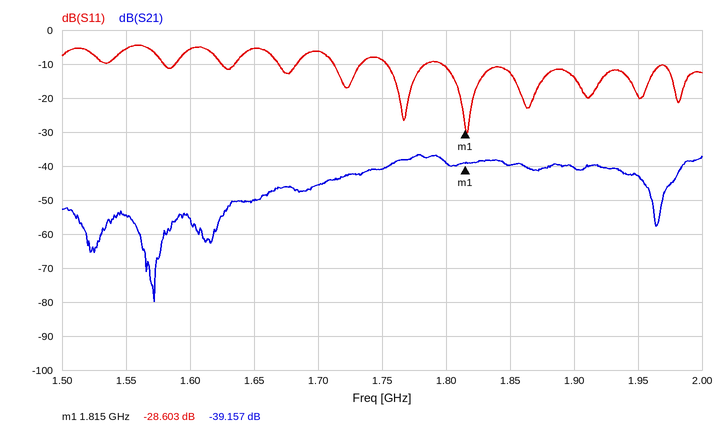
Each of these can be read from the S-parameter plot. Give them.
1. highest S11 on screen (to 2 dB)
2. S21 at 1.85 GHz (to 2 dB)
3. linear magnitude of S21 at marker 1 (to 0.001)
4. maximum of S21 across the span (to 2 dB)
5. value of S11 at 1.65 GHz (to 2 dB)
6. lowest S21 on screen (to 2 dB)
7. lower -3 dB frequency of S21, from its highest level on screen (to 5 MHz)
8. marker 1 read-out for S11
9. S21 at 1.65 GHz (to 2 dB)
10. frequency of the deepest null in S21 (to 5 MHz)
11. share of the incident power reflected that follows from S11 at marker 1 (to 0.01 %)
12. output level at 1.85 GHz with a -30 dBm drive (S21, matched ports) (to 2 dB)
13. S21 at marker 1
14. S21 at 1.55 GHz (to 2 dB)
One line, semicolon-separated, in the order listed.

-4 dB; -40 dB; 0.011; -36 dB; -6 dB; -80 dB; 1.755 GHz; -28.603 dB; -50 dB; 1.570 GHz; 0.14 %; -70 dBm; -39.157 dB; -54 dB
